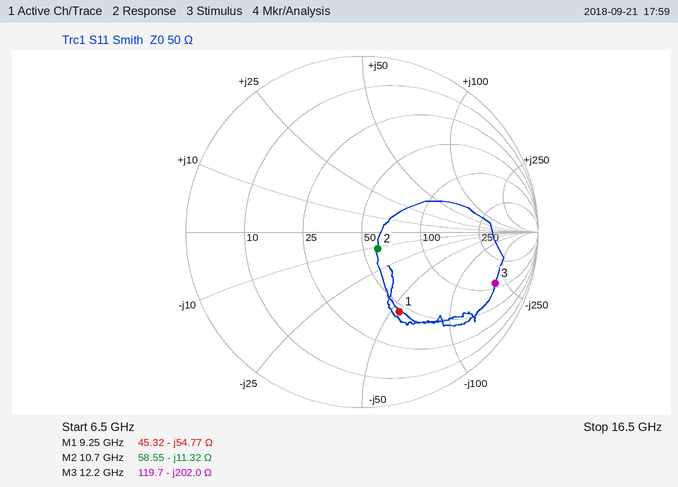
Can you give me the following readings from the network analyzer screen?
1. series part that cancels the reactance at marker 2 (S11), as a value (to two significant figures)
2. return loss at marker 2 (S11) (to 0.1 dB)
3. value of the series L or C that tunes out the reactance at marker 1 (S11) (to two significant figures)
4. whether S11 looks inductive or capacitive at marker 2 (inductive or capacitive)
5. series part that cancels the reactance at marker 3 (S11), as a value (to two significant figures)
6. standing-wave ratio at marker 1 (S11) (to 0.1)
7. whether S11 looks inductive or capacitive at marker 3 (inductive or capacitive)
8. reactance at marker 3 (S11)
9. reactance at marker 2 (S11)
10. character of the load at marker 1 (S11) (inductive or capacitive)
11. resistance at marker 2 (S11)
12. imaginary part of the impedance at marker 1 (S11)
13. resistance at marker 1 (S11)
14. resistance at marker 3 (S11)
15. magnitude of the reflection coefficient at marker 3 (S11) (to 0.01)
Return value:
170 pH
17.7 dB
940 pH
capacitive
2.6 nH
3.0
capacitive
-202.0 Ω
-11.32 Ω
capacitive
58.55 Ω
-54.77 Ω
45.32 Ω
119.7 Ω
0.81
